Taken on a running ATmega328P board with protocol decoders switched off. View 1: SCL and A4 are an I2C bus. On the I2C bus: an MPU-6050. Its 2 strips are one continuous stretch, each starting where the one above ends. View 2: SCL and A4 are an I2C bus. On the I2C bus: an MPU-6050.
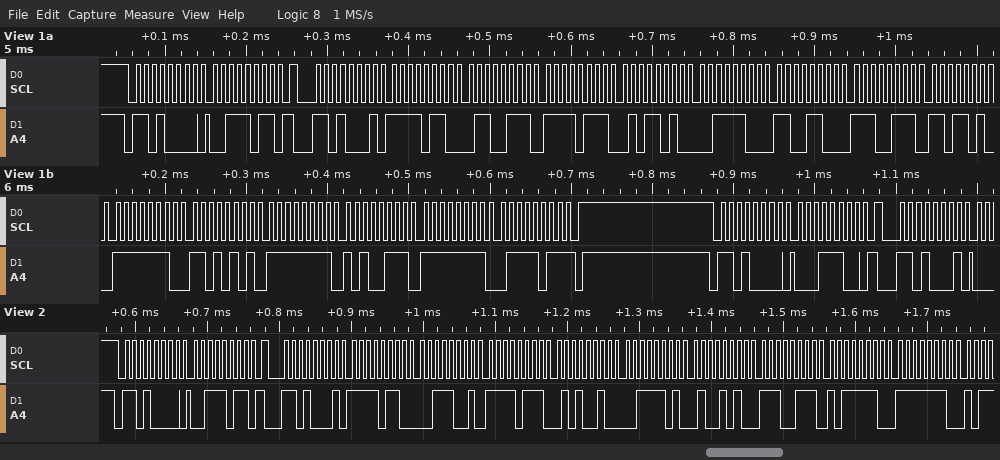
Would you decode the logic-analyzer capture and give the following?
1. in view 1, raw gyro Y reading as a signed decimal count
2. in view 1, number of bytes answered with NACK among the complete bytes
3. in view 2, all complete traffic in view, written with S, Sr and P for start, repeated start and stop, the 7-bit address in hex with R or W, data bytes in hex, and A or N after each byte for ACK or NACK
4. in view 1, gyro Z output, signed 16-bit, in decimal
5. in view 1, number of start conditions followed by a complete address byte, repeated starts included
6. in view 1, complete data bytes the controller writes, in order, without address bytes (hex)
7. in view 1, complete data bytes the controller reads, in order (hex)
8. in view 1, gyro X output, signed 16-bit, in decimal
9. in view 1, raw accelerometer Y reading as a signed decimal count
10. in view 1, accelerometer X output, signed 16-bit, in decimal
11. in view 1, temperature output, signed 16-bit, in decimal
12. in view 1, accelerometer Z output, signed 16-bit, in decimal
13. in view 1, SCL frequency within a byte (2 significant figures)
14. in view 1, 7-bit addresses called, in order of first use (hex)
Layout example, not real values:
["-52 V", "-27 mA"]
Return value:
["-89", "1", "S 68W A 3B A Sr 68R A F6 A 39 A F7 A 52 A 3D A 4A A E7 A BE A FE A", "-133", "4", "3B 1C", "F6 67 F7 5A 3C CC E7 DA FE D5 FF A7 FF 7B", "-299", "-2214", "-2457", "-6182", "15564", "100 kHz", "0x68"]
